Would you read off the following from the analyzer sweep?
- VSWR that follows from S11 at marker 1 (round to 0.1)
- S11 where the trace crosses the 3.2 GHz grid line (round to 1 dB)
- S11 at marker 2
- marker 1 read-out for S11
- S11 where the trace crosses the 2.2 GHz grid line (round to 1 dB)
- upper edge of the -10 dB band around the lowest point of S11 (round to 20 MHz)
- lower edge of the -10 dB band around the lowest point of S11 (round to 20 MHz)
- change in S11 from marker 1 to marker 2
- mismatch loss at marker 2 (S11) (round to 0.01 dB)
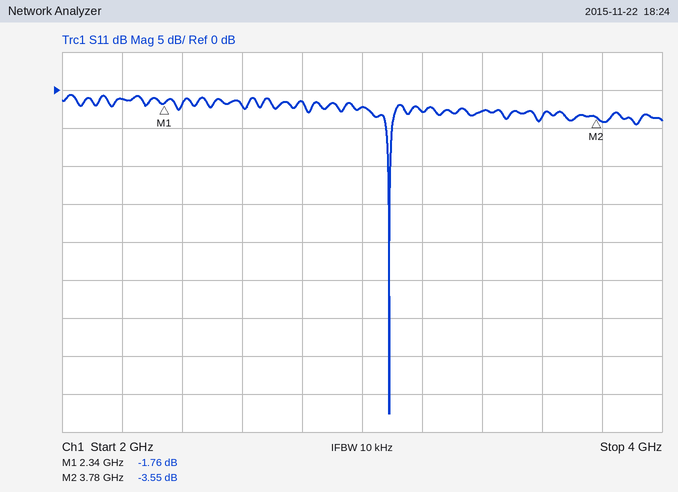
9.9
-3 dB
-3.55 dB
-1.76 dB
-1 dB
3.10 GHz
3.08 GHz
-1.79 dB
2.53 dB
